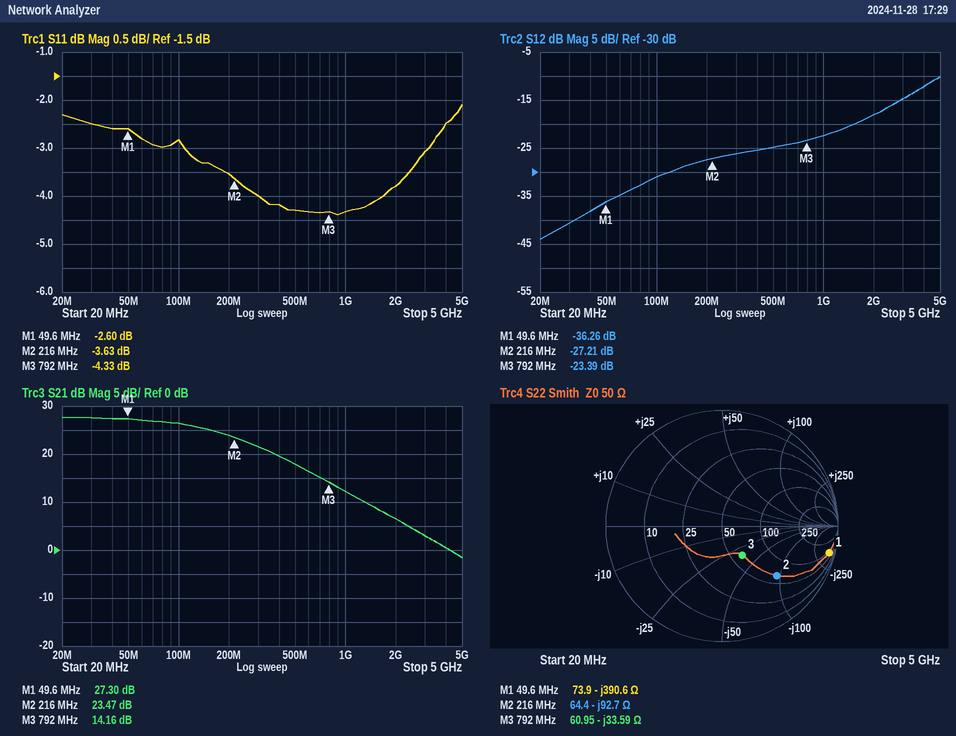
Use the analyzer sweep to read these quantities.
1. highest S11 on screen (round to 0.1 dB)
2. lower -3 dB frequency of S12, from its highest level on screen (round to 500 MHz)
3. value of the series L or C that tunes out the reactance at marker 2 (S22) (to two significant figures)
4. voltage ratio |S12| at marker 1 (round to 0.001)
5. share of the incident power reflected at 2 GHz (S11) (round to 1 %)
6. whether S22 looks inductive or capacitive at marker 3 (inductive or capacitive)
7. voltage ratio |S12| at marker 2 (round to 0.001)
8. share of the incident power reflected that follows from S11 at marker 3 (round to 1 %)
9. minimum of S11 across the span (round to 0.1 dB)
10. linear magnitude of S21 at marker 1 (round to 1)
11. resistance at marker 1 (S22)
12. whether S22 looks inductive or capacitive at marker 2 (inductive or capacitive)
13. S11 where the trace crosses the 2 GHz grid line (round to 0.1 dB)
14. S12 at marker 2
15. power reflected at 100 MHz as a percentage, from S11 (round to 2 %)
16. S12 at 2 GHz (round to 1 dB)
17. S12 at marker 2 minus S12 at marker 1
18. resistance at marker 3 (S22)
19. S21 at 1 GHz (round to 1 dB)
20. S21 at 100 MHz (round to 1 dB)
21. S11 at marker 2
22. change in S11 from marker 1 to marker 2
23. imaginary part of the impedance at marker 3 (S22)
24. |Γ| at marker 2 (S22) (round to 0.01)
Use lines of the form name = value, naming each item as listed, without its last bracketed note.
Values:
highest S11 on screen = -2.1 dB
lower -3 dB frequency of S12, from its highest level on screen = 3.5 GHz
value of the series L or C that tunes out the reactance at marker 2 (S22) = 68 nH
voltage ratio |S12| at marker 1 = 0.015
share of the incident power reflected at 2 GHz (S11) = 42 %
whether S22 looks inductive or capacitive at marker 3 = capacitive
voltage ratio |S12| at marker 2 = 0.044
share of the incident power reflected that follows from S11 at marker 3 = 37 %
minimum of S11 across the span = -4.4 dB
linear magnitude of S21 at marker 1 = 23
resistance at marker 1 = 73.9 Ω
whether S22 looks inductive or capacitive at marker 2 = capacitive
S11 where the trace crosses the 2 GHz grid line = -3.8 dB
S12 at marker 2 = -27.21 dB
power reflected at 100 MHz as a percentage, from S11 = 52 %
S12 at 2 GHz = -18 dB
S12 at marker 2 minus S12 at marker 1 = 9.05 dB
resistance at marker 3 = 60.95 Ω
S21 at 1 GHz = 12 dB
S21 at 100 MHz = 26 dB
S11 at marker 2 = -3.63 dB
change in S11 from marker 1 to marker 2 = -1.03 dB
imaginary part of the impedance at marker 3 = -33.59 Ω
|Γ| at marker 2 (S22) = 0.64
